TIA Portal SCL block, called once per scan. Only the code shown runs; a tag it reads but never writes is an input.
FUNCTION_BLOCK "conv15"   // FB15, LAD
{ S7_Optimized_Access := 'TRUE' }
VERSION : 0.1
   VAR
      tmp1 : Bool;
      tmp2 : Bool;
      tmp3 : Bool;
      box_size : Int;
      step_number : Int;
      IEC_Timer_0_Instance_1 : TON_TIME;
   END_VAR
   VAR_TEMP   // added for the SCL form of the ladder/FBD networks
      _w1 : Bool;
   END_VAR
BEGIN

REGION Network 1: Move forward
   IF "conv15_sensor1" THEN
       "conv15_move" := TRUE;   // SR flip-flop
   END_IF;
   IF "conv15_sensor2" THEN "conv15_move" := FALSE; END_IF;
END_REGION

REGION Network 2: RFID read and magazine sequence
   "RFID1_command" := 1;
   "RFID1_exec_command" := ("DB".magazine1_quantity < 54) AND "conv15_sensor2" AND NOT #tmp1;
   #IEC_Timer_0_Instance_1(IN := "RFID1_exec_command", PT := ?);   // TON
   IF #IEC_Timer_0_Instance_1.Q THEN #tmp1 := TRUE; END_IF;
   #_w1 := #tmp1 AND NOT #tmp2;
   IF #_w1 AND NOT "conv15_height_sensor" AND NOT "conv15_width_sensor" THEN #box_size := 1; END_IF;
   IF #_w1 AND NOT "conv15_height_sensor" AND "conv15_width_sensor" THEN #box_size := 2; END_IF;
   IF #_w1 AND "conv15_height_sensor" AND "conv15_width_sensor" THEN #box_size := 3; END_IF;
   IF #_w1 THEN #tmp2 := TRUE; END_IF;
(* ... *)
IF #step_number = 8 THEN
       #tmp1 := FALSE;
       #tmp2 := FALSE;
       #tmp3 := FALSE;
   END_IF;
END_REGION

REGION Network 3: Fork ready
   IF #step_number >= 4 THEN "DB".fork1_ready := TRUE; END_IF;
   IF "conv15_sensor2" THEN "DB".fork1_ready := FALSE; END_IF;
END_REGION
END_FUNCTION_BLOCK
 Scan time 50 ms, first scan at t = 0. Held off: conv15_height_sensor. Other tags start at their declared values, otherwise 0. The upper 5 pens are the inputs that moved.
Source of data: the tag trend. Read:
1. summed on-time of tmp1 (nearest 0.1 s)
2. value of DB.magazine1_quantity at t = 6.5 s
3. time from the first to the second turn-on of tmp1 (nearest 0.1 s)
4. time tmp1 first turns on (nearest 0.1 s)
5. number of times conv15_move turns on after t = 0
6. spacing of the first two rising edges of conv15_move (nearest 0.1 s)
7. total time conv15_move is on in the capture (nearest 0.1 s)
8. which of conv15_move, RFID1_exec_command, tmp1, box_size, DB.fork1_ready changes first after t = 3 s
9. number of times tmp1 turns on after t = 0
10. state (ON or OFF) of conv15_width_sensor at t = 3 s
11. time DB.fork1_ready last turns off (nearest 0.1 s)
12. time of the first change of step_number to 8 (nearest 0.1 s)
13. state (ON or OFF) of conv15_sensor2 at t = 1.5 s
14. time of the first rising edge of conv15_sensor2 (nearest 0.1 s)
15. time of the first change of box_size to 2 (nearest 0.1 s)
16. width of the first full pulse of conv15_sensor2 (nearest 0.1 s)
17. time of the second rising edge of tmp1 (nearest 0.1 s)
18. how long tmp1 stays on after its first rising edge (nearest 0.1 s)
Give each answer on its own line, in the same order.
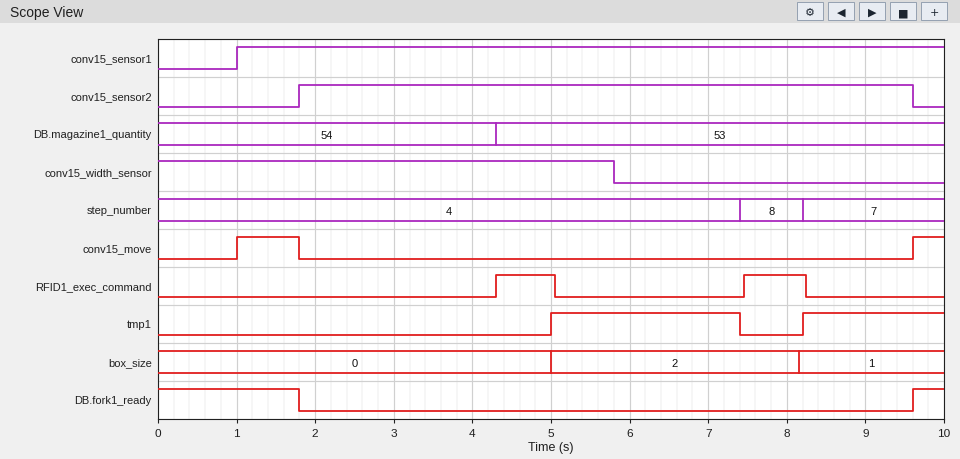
4.2 s
53
3.2 s
5.0 s
2
8.6 s
1.2 s
RFID1_exec_command
2
ON
1.8 s
7.4 s
OFF
1.8 s
5.0 s
7.8 s
8.2 s
2.4 s
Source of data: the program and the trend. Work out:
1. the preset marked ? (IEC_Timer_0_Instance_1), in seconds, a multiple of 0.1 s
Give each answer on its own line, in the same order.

0.7 s
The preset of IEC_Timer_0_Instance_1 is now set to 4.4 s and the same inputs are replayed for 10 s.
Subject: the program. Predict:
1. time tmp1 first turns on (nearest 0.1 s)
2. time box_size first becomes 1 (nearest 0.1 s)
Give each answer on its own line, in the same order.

8.7 s
8.7 s
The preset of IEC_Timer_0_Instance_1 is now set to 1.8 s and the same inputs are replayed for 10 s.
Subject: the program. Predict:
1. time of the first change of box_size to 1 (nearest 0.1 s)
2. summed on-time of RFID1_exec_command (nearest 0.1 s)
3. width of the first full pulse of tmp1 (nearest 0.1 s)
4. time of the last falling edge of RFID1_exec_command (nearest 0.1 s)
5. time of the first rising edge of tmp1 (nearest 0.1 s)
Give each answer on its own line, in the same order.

6.1 s
3.7 s
1.3 s
9.3 s
6.1 s
